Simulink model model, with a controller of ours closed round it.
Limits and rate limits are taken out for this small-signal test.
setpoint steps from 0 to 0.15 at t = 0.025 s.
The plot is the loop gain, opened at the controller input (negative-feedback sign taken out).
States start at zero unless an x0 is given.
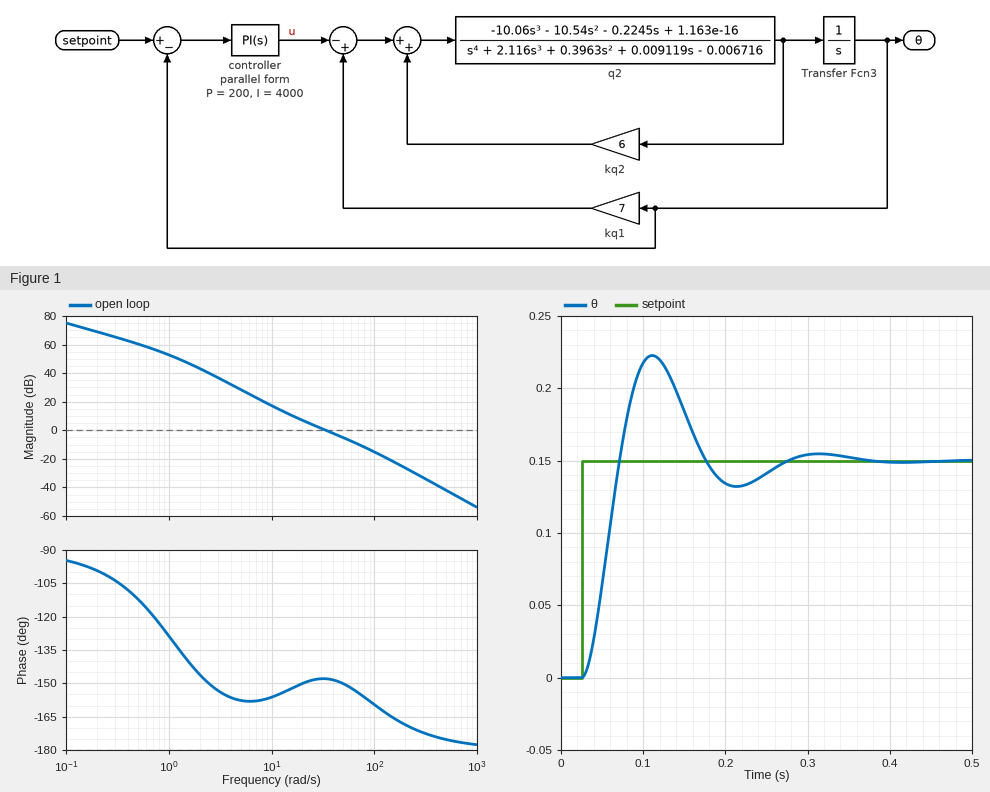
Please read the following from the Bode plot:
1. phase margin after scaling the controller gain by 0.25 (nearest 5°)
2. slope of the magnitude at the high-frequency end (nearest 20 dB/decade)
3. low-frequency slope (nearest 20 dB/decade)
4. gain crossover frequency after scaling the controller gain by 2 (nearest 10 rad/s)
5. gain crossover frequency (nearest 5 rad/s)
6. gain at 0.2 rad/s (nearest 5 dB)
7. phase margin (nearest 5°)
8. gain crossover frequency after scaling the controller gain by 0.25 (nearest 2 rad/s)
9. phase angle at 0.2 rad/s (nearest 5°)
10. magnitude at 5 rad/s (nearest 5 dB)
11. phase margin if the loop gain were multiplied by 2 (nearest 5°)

25°
-40 dB/decade
-20 dB/decade
50 rad/s
35 rad/s
70 dB
30°
14 rad/s
-100°
30 dB
30°
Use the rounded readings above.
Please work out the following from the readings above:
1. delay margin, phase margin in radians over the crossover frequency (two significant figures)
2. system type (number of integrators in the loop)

0.015 s
1
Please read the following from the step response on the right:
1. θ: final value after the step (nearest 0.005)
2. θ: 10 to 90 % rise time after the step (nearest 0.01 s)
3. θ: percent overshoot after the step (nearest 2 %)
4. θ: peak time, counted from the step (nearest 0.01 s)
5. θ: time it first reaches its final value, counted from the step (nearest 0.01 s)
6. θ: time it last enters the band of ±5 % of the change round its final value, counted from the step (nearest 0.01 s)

0.150
0.03 s
48 %
0.09 s
0.05 s
0.23 s
